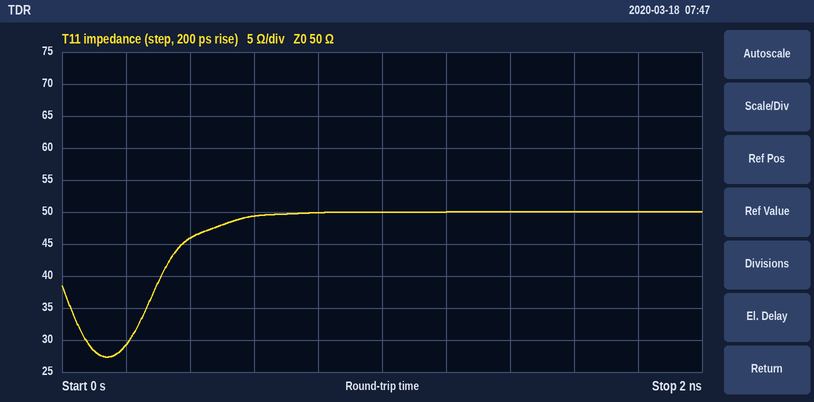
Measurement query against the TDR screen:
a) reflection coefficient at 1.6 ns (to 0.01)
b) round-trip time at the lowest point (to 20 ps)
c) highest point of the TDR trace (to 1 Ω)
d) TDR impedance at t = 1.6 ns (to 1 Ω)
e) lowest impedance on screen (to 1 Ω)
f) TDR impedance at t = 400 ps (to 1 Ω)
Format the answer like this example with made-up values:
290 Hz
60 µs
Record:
0.00
140 ps
50 Ω
50 Ω
27 Ω
46 Ω
